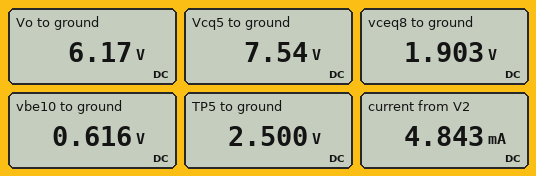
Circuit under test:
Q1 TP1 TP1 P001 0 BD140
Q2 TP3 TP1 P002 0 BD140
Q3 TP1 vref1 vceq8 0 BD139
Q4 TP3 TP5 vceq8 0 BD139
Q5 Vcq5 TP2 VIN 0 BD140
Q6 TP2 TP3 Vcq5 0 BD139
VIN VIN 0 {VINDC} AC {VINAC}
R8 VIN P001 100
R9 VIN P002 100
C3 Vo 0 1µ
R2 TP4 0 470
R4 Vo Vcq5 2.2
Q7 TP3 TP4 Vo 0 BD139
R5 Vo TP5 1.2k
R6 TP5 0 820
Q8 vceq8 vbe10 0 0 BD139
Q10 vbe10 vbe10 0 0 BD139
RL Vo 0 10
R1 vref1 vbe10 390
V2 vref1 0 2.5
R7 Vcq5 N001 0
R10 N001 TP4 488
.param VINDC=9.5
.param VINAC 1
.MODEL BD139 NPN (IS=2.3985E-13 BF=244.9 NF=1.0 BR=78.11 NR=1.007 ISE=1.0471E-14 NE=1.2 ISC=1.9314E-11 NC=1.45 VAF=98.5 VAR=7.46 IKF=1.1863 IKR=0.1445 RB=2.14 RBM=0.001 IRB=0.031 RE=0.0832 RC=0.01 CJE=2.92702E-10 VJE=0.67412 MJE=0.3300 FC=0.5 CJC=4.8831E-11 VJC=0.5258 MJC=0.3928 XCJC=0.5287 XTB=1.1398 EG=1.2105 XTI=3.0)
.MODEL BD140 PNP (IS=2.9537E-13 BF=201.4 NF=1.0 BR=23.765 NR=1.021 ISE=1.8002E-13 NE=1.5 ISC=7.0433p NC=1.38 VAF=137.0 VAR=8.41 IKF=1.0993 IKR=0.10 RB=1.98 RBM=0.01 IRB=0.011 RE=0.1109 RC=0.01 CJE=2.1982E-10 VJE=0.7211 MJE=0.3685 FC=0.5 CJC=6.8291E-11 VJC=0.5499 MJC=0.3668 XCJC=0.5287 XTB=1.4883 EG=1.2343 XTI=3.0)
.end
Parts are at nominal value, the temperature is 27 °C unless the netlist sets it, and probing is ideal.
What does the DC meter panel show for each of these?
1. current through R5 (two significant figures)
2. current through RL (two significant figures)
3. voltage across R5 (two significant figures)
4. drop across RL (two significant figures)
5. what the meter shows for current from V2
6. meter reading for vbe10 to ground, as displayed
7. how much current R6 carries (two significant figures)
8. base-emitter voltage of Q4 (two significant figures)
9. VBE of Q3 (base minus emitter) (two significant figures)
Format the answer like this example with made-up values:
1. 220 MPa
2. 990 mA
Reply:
1. 3.1 mA
2. 620 mA
3. 3.7 V
4. 6.2 V
5. 4.843 mA
6. 0.616 V
7. 3.0 mA
8. 600 mV
9. 600 mV
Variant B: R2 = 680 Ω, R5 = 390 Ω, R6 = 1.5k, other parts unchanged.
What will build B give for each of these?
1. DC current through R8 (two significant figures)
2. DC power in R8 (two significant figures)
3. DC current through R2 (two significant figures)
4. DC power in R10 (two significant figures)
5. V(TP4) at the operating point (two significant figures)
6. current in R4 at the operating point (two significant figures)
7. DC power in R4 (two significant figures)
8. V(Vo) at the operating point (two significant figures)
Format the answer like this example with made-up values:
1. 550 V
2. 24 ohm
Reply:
1. 2.4 mA
2. 580 µW
3. 3.3 mA
4. 5.3 mW
5. 2.2 V
6. 320 mA
7. 220 mW
8. 3.2 V
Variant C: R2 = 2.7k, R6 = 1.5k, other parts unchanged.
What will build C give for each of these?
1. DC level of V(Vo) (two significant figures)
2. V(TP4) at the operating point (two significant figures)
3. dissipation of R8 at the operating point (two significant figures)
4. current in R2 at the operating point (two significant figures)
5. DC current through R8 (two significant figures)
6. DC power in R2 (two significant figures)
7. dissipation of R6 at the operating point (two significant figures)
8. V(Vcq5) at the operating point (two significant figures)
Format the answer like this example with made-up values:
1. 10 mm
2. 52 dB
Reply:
1. 4.5 V
2. 4.7 V
3. 580 µW
4. 1.7 mA
5. 2.4 mA
6. 8.1 mW
7. 4.2 mW
8. 5.5 V
